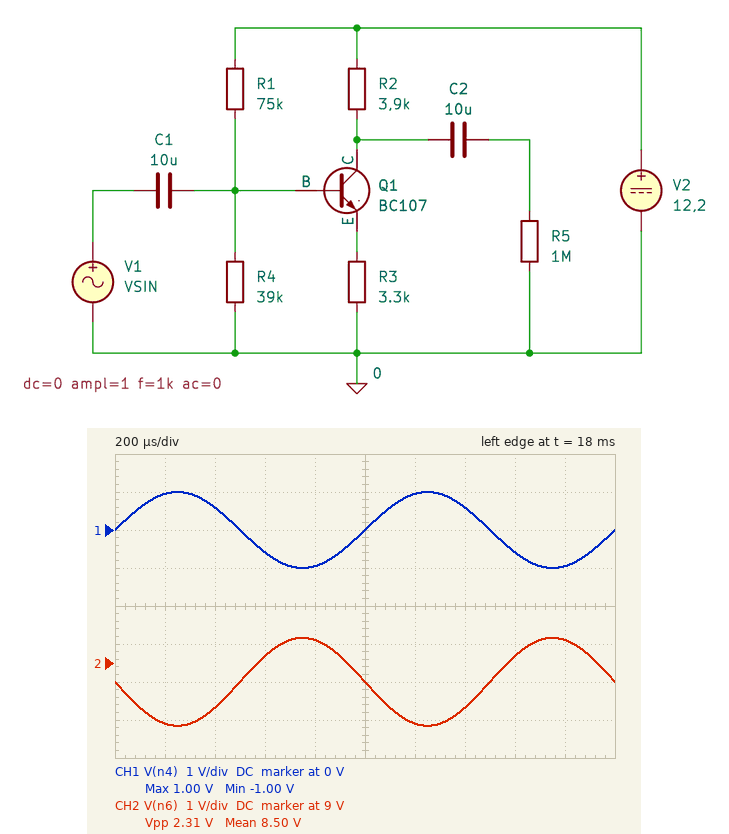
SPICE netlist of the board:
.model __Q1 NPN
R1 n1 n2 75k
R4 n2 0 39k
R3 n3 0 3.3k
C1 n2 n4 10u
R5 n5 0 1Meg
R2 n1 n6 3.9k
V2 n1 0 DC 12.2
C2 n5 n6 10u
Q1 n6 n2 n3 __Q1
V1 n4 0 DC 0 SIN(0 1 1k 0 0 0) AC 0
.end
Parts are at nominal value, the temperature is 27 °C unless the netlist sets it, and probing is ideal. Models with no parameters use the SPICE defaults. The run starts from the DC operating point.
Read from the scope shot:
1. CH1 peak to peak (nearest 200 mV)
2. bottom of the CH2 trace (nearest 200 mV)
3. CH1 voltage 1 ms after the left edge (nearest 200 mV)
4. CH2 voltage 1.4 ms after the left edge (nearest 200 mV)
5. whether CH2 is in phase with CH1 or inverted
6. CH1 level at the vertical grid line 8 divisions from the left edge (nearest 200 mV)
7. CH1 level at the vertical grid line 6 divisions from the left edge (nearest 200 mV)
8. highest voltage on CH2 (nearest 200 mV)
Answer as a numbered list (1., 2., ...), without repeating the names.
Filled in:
1. 2.0 V
2. 7.4 V
3. 0 V
4. 7.8 V
5. inverted
6. -600 mV
7. 1.0 V
8. 9.6 V
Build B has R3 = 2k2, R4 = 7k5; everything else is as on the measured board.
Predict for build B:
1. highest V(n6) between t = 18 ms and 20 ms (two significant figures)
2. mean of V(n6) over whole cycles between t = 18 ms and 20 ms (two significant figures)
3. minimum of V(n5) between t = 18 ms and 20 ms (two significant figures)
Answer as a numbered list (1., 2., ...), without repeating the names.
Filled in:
1. 12 V
2. 11 V
3. -1.7 V
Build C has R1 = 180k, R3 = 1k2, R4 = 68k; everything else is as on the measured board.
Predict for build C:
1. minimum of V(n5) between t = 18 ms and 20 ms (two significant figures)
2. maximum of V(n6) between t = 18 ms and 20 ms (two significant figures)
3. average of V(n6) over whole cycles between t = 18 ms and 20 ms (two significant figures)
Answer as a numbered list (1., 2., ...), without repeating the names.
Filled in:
1. -3.2 V
2. 9.5 V
3. 6.3 V
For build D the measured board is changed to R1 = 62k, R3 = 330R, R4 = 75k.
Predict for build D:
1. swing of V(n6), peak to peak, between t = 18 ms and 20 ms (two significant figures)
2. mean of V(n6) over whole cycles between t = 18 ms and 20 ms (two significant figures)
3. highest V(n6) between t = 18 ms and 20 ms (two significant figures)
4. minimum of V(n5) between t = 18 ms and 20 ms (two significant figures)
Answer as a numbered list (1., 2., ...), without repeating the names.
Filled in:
1. 11 V
2. 7.0 V
3. 12 V
4. -13 mV
